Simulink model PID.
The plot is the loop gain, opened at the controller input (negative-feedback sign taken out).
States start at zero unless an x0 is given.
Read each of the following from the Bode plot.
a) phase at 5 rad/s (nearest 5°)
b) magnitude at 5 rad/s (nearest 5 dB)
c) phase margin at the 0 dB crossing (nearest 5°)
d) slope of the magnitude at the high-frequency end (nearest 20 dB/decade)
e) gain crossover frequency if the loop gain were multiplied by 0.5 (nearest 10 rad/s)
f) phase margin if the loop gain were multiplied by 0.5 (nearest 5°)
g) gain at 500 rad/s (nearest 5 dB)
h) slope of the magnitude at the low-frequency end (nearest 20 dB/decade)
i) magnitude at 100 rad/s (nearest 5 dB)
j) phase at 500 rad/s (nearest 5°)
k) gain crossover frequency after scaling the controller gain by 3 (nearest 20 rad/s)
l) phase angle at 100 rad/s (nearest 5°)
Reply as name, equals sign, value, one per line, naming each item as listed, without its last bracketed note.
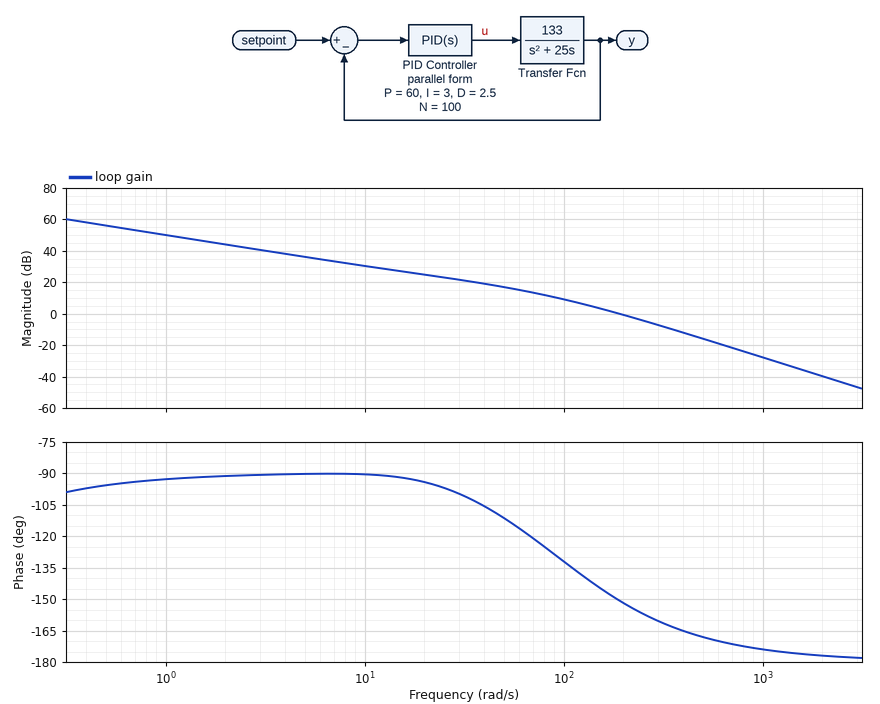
phase at 5 rad/s = -90°
magnitude at 5 rad/s = 35 dB
phase margin at the 0 dB crossing = 30°
slope of the magnitude at the high-frequency end = -40 dB/decade
gain crossover frequency if the loop gain were multiplied by 0.5 = 130 rad/s
phase margin if the loop gain were multiplied by 0.5 = 40°
gain at 500 rad/s = -15 dB
slope of the magnitude at the low-frequency end = -20 dB/decade
magnitude at 100 rad/s = 10 dB
phase at 500 rad/s = -170°
gain crossover frequency after scaling the controller gain by 3 = 340 rad/s
phase angle at 100 rad/s = -130°
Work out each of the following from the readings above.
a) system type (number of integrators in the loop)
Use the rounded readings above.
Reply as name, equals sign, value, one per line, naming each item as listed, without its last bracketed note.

system type = 1
